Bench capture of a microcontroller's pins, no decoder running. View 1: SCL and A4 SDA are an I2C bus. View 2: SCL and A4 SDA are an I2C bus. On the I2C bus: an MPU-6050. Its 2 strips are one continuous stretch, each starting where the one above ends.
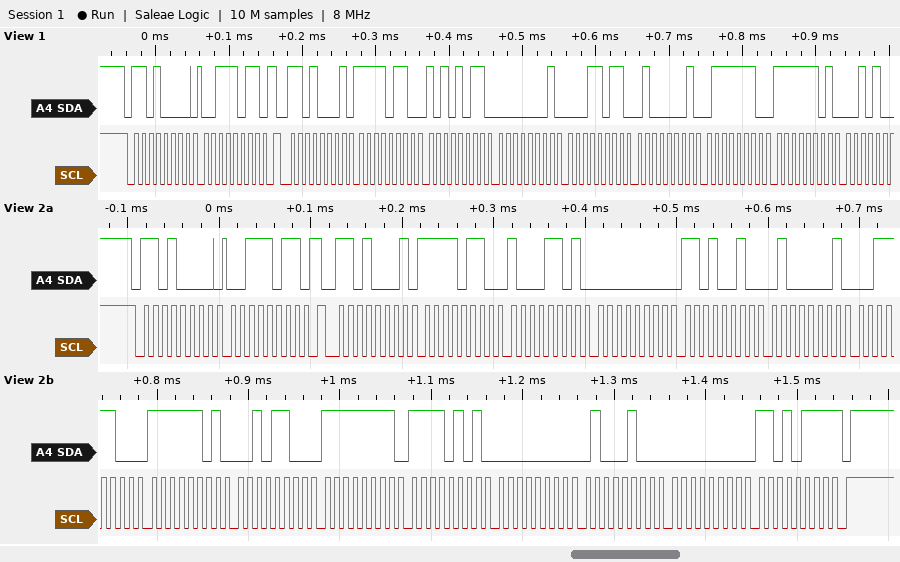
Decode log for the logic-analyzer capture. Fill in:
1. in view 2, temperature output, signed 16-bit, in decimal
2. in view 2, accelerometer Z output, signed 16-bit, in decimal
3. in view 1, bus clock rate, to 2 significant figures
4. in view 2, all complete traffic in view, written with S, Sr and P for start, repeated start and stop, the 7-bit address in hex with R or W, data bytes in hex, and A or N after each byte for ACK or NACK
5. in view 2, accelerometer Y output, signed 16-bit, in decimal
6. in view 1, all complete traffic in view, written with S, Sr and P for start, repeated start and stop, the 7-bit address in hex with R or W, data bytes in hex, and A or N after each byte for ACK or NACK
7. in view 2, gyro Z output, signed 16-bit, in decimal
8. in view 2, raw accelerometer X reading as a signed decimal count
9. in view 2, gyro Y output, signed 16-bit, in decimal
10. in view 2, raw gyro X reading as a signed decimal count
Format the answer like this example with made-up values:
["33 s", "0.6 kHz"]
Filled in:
["-724", "16700", "100 kHz", "S 68W A 3B A Sr 68R A F6 A 8D A 00 A D2 A 41 A 3C A FD A 2C A FF A F5 A 00 A 44 A 00 A D7 N P", "210", "S 68W A 3B A Sr 68R A F6 A AB A 01 A 1B A 41 A 7E A FD A", "215", "-2419", "68", "-11"]
